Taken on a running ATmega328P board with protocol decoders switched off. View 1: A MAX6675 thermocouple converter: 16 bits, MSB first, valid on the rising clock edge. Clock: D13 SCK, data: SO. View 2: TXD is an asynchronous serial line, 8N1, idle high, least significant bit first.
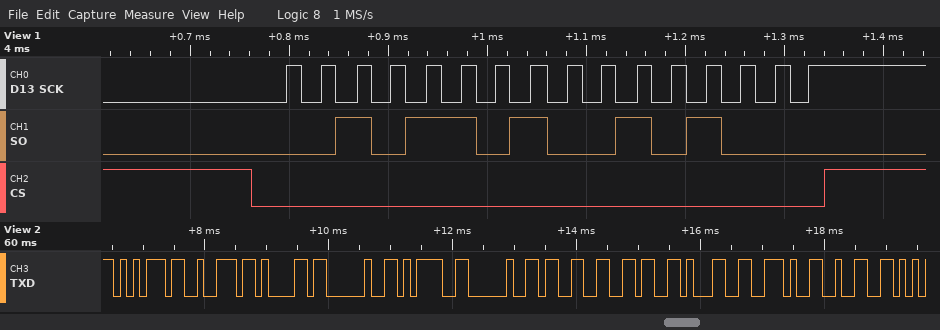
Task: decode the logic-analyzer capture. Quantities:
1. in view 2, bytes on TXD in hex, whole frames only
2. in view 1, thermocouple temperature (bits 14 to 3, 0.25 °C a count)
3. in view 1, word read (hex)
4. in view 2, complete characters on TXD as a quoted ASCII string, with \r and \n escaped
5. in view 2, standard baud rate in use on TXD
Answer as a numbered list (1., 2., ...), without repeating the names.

1. 0x75 0x72 0x61 0x20 0x3D 0x20 0x33 0x36 0x31 0x2E 0x32
2. 361.25 °C
3. 0x2D28
4. "ura = 361.2"
5. 9600 baud
